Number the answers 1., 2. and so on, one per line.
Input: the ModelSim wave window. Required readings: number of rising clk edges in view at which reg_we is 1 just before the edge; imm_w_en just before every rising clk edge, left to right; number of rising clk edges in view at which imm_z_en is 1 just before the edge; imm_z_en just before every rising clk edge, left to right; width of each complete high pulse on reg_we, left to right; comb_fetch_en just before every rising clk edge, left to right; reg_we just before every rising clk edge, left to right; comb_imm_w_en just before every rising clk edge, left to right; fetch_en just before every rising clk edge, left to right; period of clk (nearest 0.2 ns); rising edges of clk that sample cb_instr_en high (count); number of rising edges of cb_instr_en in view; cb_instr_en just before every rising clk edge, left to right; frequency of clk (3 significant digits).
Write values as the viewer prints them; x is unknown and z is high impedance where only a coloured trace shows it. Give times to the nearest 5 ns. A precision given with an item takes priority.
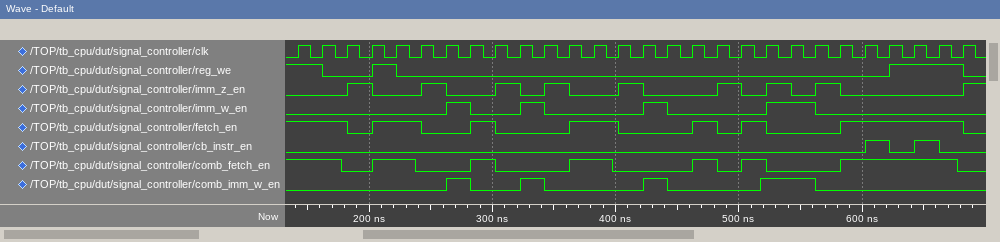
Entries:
1. 6
2. 0 0 0 0 0 0 0 1 0 0 1 0 0 0 0 1 0 0 0 0 1 1 0 0 0 0 0 0
3. 8
4. 0 0 0 1 0 0 1 0 0 1 0 1 0 0 1 0 0 0 1 0 1 0 1 0 0 0 0 0
5. 20 ns, 60 ns
6. 1 1 0 0 1 0 0 0 1 0 0 0 1 0 0 0 0 1 0 1 0 0 0 1 1 1 1 0
7. 1 1 0 0 1 0 0 0 0 0 0 0 0 0 0 0 0 0 0 0 0 0 0 0 0 1 1 1
8. 0 0 0 0 0 0 0 1 0 0 1 0 0 0 0 1 0 0 0 1 1 1 0 0 0 0 0 0
9. 1 1 1 0 1 1 0 0 1 0 0 0 1 1 0 0 0 1 0 1 0 0 0 1 1 1 1 1
10. 20 ns
11. 2
12. 2
13. 0 0 0 0 0 0 0 0 0 0 0 0 0 0 0 0 0 0 0 0 0 0 0 0 1 0 1 0
14. 50.0 MHz
